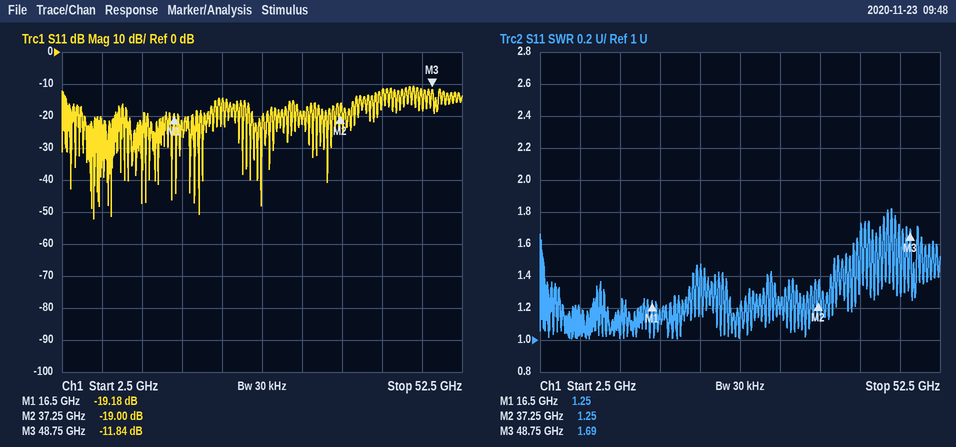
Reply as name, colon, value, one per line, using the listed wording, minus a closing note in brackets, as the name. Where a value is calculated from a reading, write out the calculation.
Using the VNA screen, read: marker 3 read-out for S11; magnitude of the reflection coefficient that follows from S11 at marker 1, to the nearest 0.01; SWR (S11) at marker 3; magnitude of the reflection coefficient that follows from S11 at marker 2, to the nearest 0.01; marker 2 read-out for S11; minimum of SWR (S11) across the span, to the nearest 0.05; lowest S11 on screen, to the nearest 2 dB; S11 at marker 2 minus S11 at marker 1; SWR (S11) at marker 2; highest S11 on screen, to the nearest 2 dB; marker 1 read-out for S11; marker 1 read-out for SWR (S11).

marker 3 read-out for S11: -11.84 dB
magnitude of the reflection coefficient that follows from S11 at marker 1, to the nearest 0.01: 10^(-19.18/20) ≈ 0.11
SWR (S11) at marker 3: 1.69
magnitude of the reflection coefficient that follows from S11 at marker 2, to the nearest 0.01: 10^(-19/20) ≈ 0.11
marker 2 read-out for S11: -19.00 dB
minimum of SWR (S11) across the span, to the nearest 0.05: 1.00
lowest S11 on screen, to the nearest 2 dB: -52 dB
S11 at marker 2 minus S11 at marker 1: -19 − (-19.18) = 0.18 dB
SWR (S11) at marker 2: 1.25
highest S11 on screen, to the nearest 2 dB: -10 dB
marker 1 read-out for S11: -19.18 dB
marker 1 read-out for SWR: 1.25
